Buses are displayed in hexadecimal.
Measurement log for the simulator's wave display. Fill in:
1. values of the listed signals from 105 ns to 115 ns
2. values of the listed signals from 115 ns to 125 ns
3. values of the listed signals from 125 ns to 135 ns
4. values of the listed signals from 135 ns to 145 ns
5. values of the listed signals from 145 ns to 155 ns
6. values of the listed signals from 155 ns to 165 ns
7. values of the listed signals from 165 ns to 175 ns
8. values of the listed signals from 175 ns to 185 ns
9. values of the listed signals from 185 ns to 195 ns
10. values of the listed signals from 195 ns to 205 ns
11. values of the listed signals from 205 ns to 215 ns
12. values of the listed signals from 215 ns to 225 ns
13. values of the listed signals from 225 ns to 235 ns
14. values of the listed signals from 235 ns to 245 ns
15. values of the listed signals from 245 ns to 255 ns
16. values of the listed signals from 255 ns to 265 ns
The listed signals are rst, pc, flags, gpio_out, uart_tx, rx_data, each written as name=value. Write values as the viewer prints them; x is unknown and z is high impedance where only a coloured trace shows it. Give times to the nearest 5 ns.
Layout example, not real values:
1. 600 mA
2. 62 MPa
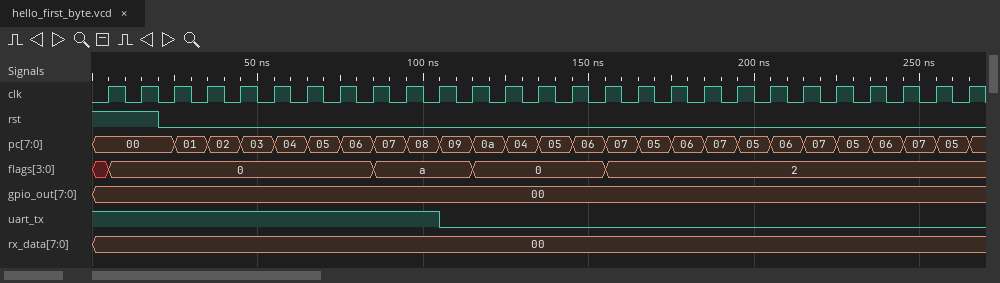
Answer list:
1. rst=0, pc=09, flags=a, gpio_out=00, uart_tx=0, rx_data=00
2. rst=0, pc=0a, flags=0, gpio_out=00, uart_tx=0, rx_data=00
3. rst=0, pc=04, flags=0, gpio_out=00, uart_tx=0, rx_data=00
4. rst=0, pc=05, flags=0, gpio_out=00, uart_tx=0, rx_data=00
5. rst=0, pc=06, flags=0, gpio_out=00, uart_tx=0, rx_data=00
6. rst=0, pc=07, flags=2, gpio_out=00, uart_tx=0, rx_data=00
7. rst=0, pc=05, flags=2, gpio_out=00, uart_tx=0, rx_data=00
8. rst=0, pc=06, flags=2, gpio_out=00, uart_tx=0, rx_data=00
9. rst=0, pc=07, flags=2, gpio_out=00, uart_tx=0, rx_data=00
10. rst=0, pc=05, flags=2, gpio_out=00, uart_tx=0, rx_data=00
11. rst=0, pc=06, flags=2, gpio_out=00, uart_tx=0, rx_data=00
12. rst=0, pc=07, flags=2, gpio_out=00, uart_tx=0, rx_data=00
13. rst=0, pc=05, flags=2, gpio_out=00, uart_tx=0, rx_data=00
14. rst=0, pc=06, flags=2, gpio_out=00, uart_tx=0, rx_data=00
15. rst=0, pc=07, flags=2, gpio_out=00, uart_tx=0, rx_data=00
16. rst=0, pc=05, flags=2, gpio_out=00, uart_tx=0, rx_data=00
